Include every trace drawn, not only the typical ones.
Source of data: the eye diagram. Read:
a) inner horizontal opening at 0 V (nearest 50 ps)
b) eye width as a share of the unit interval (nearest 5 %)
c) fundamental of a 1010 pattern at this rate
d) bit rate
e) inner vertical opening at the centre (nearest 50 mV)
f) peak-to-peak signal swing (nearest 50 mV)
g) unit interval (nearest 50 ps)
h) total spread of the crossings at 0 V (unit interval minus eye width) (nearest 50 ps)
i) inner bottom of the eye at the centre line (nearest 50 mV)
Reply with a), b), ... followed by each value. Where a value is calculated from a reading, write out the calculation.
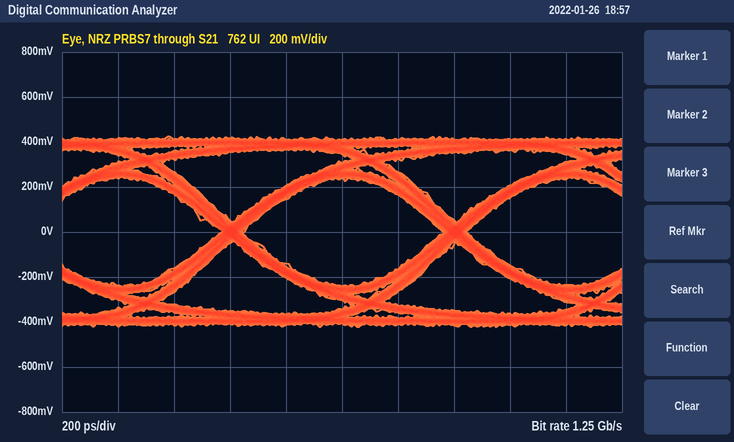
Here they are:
a) 700 ps
b) 700 ps / 800 ps ≈ 87.5 %, so 90 % to the nearest 5 %
c) 625 MHz
d) 1.25 Gb/s
e) 500 mV
f) 850 mV
g) 800 ps
h) 100 ps
i) -250 mV
